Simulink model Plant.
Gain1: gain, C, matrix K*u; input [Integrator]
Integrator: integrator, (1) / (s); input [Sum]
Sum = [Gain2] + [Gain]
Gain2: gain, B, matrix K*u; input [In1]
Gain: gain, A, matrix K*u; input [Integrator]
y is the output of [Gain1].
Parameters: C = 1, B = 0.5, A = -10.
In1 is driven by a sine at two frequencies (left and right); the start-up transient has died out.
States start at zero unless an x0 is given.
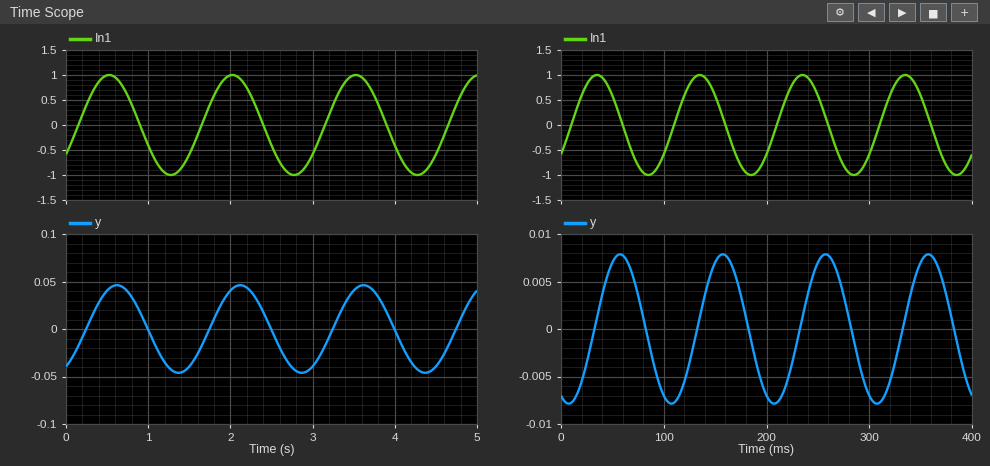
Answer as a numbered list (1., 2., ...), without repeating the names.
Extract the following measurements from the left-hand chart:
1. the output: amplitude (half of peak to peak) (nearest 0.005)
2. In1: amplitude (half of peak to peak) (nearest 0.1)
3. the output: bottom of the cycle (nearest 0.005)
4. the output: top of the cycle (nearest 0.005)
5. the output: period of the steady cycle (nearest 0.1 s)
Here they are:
1. 0.045
2. 1.0
3. -0.045
4. 0.045
5. 1.5 s
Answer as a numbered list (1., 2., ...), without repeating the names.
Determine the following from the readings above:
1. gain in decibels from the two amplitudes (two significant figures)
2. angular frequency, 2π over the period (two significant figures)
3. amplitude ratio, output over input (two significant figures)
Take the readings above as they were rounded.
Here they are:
1. -27 dB
2. 4.2 rad/s
3. 0.045
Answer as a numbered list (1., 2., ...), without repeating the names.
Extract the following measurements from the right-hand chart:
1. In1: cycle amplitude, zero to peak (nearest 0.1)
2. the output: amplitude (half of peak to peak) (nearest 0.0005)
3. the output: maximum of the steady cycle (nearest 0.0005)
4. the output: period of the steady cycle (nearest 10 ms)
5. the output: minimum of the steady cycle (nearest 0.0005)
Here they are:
1. 1.0
2. 0.0080
3. 0.0080
4. 100 ms
5. -0.0080
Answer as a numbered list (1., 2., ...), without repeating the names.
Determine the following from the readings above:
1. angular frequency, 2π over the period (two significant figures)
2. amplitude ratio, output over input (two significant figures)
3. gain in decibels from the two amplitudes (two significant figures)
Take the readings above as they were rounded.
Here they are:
1. 0.063 rad/ms
2. 0.0080
3. -42 dB
